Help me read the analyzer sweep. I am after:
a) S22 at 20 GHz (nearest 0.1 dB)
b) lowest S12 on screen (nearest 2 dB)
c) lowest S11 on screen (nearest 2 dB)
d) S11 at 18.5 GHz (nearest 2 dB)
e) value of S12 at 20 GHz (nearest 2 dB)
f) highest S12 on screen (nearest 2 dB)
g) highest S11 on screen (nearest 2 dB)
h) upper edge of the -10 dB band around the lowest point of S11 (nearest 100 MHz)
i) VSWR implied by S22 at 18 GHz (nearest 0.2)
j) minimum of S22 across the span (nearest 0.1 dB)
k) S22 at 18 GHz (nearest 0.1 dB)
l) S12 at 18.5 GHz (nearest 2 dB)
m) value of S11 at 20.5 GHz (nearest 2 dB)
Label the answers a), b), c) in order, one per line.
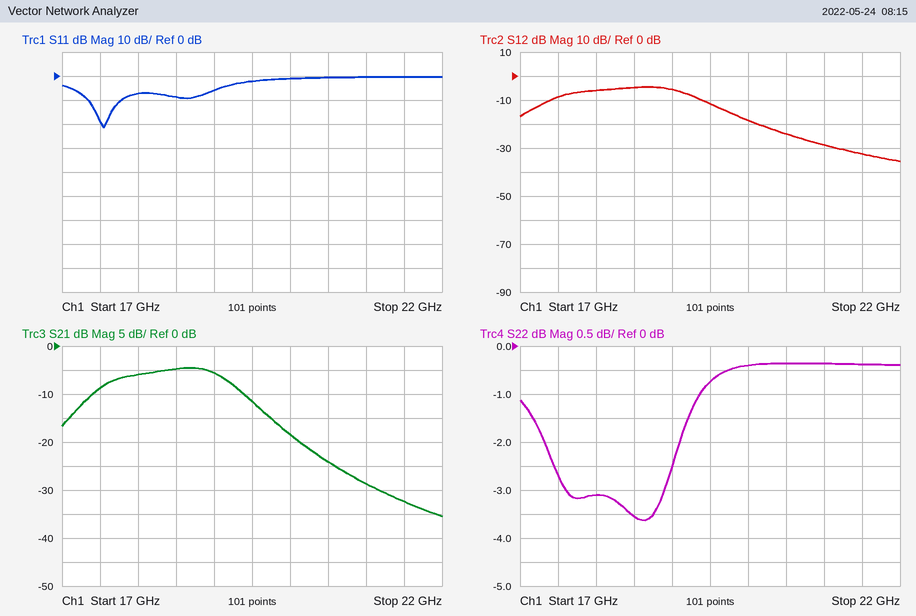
a) -0.4 dB
b) -36 dB
c) -22 dB
d) -8 dB
e) -18 dB
f) -4 dB
g) 0 dB
h) 17.8 GHz
i) 5.6
j) -3.6 dB
k) -3.1 dB
l) -4 dB
m) 0 dB
